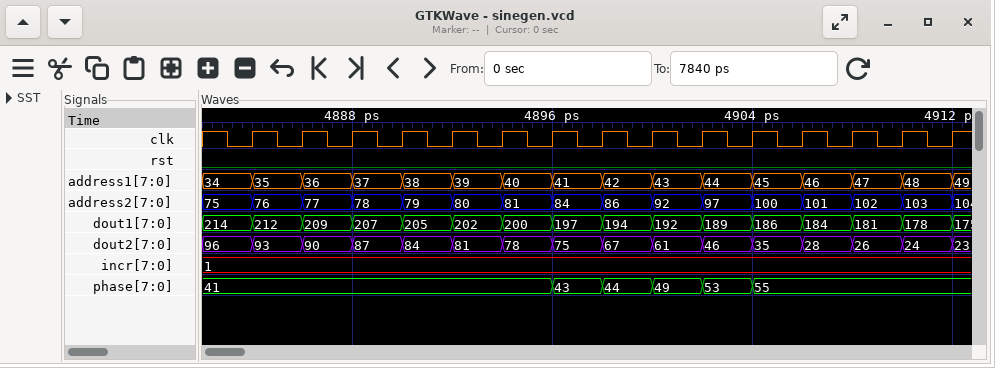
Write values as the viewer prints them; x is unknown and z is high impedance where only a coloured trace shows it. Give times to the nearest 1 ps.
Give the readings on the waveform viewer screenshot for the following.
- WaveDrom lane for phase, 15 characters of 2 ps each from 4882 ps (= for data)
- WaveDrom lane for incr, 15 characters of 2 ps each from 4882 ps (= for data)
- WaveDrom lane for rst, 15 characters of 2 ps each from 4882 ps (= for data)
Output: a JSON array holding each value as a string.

["{name: 'phase', wave: '=......=====...', data: '41 43 44 49 53 55'}", "{name: 'incr', wave: '=..............', data: '1'}", "{name: 'rst', wave: '0..............'}"]
